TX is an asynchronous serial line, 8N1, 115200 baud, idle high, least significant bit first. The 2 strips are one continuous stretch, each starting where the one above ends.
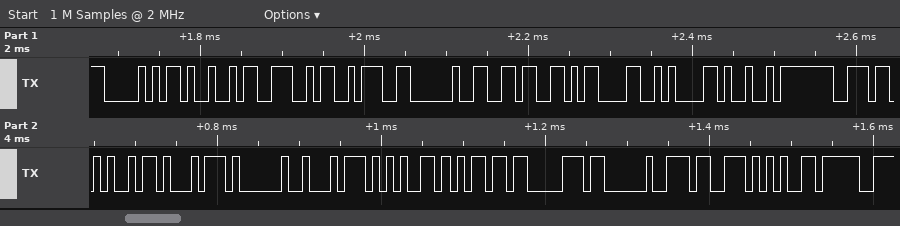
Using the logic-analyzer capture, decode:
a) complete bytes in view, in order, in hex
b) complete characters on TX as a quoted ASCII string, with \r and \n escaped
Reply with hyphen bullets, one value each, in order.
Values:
- 50 49 4E 3A 20 36 0D 0A 49 6E 69 74 20 74 65 6D 70 20 73 65
- "PIN: 6\r\nInit temp se"
